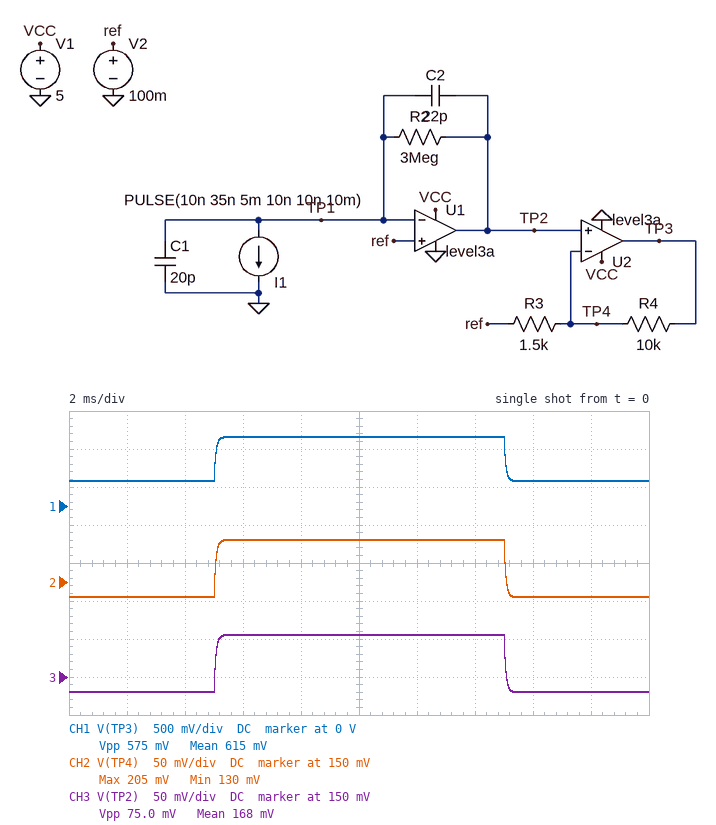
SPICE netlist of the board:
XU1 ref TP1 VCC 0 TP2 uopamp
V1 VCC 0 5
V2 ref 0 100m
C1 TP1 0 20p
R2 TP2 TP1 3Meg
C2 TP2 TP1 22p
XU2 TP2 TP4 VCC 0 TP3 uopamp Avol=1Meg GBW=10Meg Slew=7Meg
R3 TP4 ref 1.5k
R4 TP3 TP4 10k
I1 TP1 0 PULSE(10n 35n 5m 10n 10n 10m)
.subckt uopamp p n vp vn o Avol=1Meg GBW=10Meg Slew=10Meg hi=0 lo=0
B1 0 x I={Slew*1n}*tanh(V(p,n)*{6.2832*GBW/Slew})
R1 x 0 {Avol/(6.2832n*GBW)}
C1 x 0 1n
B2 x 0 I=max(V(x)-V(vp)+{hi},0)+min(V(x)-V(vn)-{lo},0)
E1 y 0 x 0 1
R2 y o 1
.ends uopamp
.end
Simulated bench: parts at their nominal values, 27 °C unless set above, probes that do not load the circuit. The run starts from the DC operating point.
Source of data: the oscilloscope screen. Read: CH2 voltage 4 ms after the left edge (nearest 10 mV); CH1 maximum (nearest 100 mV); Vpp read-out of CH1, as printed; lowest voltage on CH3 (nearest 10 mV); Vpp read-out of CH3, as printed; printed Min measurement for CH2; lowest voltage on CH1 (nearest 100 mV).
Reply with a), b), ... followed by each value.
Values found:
a) 130 mV
b) 900 mV
c) 575 mV
d) 130 mV
e) 75.0 mV
f) 130 mV
g) 300 mV
